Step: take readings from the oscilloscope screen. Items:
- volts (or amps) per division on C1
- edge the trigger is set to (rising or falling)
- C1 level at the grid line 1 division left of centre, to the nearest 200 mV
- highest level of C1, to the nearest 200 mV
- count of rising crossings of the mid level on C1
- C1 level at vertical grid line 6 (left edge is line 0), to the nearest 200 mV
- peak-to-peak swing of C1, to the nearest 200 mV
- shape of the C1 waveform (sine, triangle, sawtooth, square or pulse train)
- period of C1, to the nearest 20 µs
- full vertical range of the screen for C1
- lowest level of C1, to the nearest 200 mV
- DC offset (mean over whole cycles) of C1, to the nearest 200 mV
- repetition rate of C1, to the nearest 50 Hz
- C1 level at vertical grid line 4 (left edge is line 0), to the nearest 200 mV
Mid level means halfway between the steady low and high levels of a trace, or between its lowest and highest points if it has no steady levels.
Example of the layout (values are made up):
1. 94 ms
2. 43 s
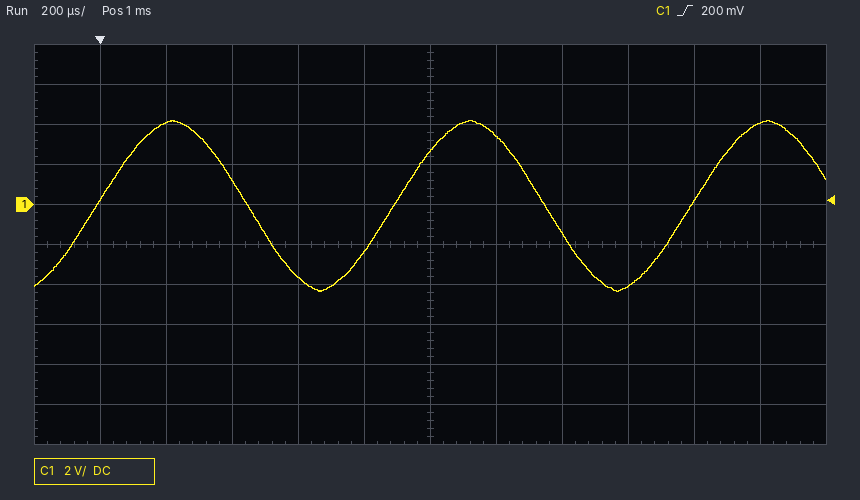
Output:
1. 2 V
2. rising
3. -2.4 V
4. 4.2 V
5. 3
6. 2.6 V
7. 8.6 V
8. sine
9. 900 µs
10. 20 V
11. -4.4 V
12. 0.0 V
13. 1.10 kHz
14. -3.6 V
